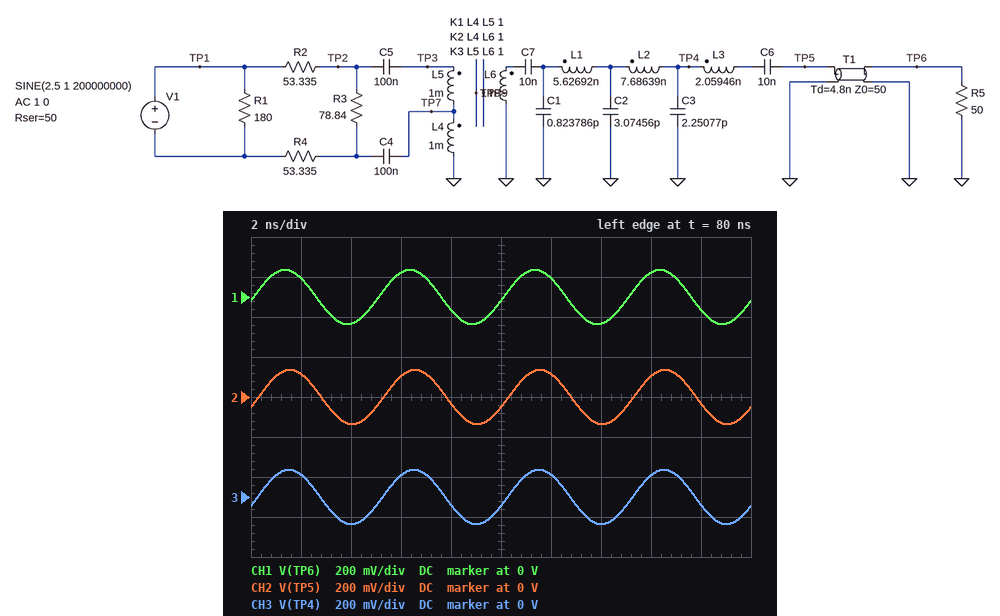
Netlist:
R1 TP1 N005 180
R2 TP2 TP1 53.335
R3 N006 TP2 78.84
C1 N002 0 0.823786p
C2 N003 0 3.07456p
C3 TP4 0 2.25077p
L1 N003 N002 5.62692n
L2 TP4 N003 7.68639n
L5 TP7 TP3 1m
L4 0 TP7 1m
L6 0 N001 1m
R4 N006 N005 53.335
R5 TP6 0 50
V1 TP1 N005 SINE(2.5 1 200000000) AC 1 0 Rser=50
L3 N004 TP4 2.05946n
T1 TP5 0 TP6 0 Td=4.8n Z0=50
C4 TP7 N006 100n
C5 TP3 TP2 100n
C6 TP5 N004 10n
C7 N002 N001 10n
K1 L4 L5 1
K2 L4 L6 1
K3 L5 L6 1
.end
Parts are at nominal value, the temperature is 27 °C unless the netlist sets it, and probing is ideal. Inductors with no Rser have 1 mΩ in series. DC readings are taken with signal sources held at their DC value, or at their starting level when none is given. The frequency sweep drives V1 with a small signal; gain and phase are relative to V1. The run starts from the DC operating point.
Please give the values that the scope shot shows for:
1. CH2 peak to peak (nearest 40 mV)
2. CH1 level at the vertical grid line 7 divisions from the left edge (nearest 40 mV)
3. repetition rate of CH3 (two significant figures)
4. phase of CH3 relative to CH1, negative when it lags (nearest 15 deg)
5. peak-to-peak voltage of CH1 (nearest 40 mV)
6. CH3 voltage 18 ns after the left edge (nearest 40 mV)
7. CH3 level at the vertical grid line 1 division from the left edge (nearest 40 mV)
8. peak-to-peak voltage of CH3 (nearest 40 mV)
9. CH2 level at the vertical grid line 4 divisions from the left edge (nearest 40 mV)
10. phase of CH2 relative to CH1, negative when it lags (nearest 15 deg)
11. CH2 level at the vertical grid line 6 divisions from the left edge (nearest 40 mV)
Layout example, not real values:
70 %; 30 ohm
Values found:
280 mV; -120 mV; 200 MHz; -15 deg; 280 mV; -40 mV; 120 mV; 280 mV; -40 mV; -15 deg; 120 mV
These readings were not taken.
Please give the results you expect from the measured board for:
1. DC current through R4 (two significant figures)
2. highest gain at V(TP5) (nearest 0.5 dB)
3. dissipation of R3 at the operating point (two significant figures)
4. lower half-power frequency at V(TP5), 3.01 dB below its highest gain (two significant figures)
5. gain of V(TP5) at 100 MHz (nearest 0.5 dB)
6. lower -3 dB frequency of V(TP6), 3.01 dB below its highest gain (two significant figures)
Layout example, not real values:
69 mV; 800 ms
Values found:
8.7 mA; -17.5 dB; 6.0 mW; 340 kHz; -17.5 dB; 340 kHz
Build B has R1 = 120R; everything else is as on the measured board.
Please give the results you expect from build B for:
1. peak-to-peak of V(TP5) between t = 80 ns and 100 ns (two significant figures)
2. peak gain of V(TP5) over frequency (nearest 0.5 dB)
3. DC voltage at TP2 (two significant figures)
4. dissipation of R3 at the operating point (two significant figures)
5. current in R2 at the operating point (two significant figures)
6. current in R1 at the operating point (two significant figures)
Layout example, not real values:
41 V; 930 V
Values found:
250 mV; -18.0 dB; 320 mV; 5.0 mW; 8.0 mA; 12 mA
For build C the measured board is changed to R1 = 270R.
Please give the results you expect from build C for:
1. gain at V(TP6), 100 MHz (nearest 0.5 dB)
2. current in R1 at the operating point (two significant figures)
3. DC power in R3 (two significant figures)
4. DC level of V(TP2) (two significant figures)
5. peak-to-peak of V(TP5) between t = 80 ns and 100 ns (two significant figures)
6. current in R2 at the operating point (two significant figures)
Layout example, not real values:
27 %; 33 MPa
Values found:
-17.0 dB; 6.4 mA; 6.8 mW; 370 mV; 290 mV; 9.3 mA
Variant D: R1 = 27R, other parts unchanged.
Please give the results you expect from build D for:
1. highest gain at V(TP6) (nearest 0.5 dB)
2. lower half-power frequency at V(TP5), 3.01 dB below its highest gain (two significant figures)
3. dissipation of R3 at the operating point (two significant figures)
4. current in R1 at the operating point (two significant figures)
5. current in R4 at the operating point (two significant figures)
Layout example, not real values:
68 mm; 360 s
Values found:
-23.0 dB; 350 kHz; 1.5 mW; 30 mA; 4.3 mA
